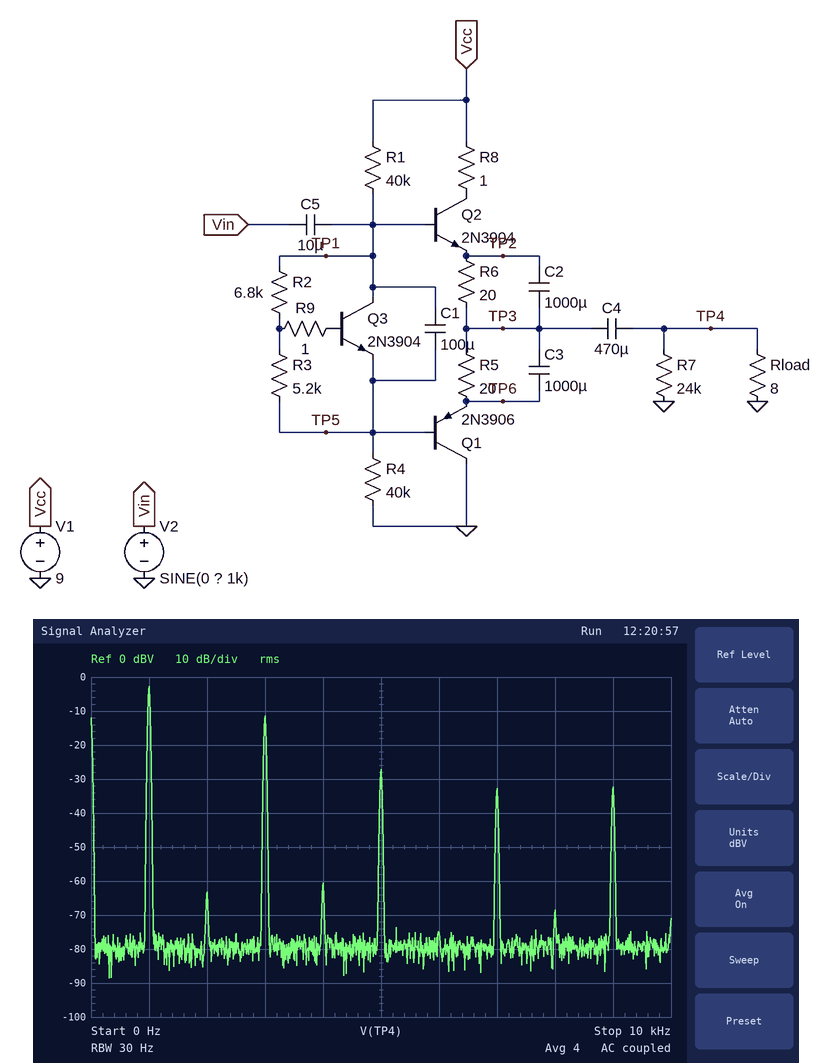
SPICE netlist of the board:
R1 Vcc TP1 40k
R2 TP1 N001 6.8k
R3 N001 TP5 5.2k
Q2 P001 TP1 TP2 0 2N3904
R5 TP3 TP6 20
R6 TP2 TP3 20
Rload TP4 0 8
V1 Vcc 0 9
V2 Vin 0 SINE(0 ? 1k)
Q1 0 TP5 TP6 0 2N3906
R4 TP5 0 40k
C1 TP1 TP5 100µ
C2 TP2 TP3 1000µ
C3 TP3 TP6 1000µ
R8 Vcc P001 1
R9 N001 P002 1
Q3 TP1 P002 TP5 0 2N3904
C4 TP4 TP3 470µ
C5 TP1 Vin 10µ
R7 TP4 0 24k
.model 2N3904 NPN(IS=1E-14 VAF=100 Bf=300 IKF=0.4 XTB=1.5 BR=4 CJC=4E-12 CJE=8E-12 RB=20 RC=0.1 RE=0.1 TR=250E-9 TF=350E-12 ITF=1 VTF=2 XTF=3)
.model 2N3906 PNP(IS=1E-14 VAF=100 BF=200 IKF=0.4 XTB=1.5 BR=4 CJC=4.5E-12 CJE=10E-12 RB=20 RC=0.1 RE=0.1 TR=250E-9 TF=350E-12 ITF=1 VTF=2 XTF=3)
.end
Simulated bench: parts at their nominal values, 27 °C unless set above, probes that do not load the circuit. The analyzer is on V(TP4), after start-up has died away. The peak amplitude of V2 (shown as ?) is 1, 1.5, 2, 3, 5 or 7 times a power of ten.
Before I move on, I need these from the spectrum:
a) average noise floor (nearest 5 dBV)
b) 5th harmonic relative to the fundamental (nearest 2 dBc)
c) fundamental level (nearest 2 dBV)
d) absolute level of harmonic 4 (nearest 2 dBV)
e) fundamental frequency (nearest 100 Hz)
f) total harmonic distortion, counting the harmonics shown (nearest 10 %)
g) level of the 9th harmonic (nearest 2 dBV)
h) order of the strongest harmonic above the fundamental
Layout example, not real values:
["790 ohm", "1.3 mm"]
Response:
["-80 dBV", "-24 dBc", "-2 dBV", "-60 dBV", "1.0 kHz", "40 %", "-32 dBV", "3"]
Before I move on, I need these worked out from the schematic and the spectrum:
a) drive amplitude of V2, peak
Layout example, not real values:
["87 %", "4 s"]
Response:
["3 V"]
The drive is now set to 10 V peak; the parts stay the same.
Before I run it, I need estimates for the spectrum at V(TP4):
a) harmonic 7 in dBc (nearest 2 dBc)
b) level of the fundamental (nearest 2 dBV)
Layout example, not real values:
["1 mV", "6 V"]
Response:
["-18 dBc", "4 dBV"]
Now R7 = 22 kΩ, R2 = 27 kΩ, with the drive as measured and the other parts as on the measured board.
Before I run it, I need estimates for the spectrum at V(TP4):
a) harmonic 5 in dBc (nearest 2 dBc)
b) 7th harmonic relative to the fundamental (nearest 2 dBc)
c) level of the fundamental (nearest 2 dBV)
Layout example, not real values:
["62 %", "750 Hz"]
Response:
["-24 dBc", "-34 dBc", "-2 dBV"]
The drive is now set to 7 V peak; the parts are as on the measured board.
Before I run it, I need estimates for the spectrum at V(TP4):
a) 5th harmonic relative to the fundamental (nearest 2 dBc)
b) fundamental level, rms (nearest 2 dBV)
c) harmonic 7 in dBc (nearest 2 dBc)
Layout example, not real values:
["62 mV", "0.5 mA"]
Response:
["-20 dBc", "4 dBV", "-24 dBc"]
